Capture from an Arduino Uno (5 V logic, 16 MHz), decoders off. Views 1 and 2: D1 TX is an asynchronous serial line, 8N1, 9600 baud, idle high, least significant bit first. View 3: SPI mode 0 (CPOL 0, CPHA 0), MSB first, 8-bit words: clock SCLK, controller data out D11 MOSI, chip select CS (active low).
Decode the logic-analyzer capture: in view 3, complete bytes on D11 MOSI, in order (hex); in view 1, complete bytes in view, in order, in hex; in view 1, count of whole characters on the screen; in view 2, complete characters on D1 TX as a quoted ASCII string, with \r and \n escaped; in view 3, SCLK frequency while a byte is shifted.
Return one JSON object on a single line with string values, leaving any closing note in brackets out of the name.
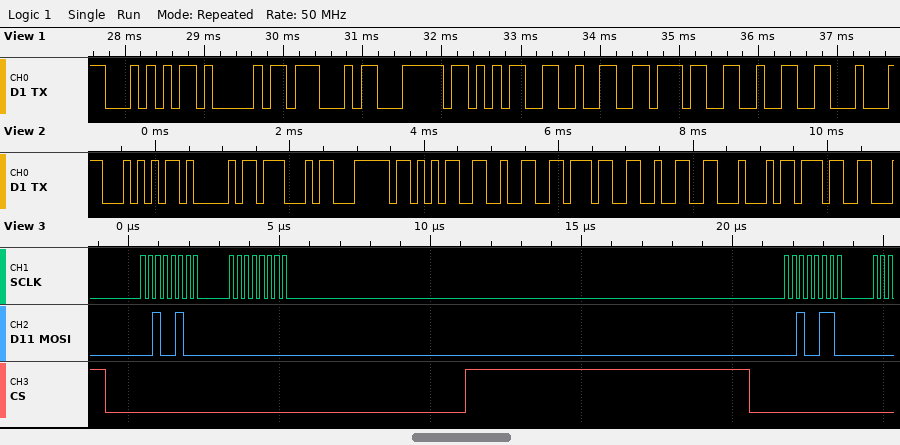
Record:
{"in view 3, complete bytes on D11 MOSI, in order": "24 00 26", "in view 1, complete bytes in view, in order, in hex": "0x54 0x41 0x47 0x7C 0x35 0x32 0x37 0x32", "in view 1, count of whole characters on the screen": "8", "in view 2, complete characters on D1 TX as a quoted ASCII string, with \\r and \\n escaped": "\"TAG|5272D7\"", "in view 3, SCLK frequency while a byte is shifted": "4 MHz"}
